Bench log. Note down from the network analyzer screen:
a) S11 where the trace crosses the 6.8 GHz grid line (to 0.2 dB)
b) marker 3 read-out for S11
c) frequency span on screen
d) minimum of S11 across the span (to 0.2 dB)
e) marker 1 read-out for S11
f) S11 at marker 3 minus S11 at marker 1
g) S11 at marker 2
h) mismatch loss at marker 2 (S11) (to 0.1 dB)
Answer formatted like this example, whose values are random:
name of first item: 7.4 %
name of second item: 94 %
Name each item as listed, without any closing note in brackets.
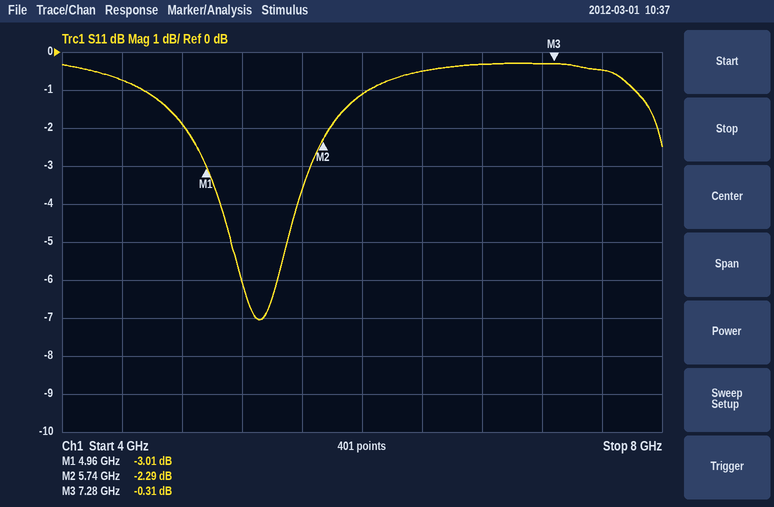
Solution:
S11 where the trace crosses the 6.8 GHz grid line: -0.4 dB
marker 3 read-out for S11: -0.31 dB
frequency span on screen: 4 GHz
minimum of S11 across the span: -7.0 dB
marker 1 read-out for S11: -3.01 dB
S11 at marker 3 minus S11 at marker 1: 2.70 dB
S11 at marker 2: -2.29 dB
mismatch loss at marker 2 (S11): 3.9 dB
